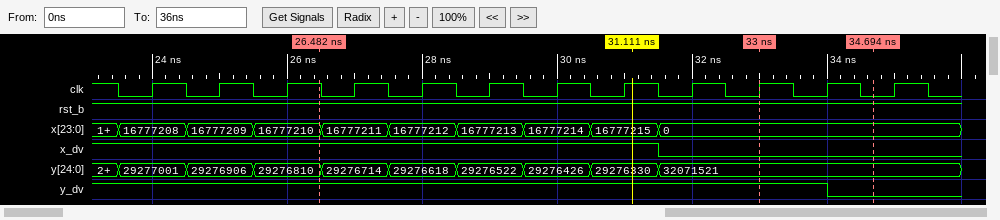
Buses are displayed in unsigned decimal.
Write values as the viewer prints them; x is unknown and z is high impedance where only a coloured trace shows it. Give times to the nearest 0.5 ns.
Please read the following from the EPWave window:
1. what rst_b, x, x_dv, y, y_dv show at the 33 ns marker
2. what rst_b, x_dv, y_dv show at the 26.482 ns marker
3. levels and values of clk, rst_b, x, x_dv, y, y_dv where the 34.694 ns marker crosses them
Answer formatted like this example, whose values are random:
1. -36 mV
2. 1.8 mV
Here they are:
1. rst_b=1, x=0, x_dv=0, y=32071521, y_dv=1
2. rst_b=1, x_dv=1, y_dv=1
3. clk=0, rst_b=1, x=0, x_dv=0, y=32071521, y_dv=0
